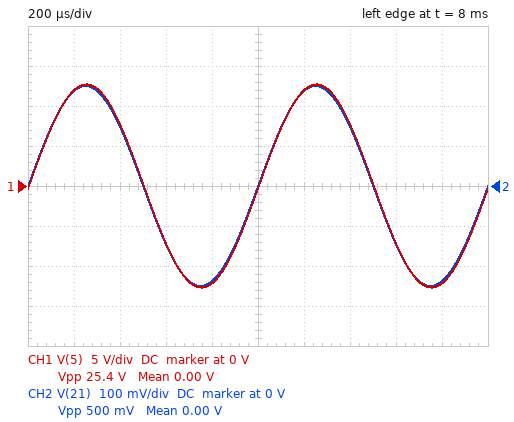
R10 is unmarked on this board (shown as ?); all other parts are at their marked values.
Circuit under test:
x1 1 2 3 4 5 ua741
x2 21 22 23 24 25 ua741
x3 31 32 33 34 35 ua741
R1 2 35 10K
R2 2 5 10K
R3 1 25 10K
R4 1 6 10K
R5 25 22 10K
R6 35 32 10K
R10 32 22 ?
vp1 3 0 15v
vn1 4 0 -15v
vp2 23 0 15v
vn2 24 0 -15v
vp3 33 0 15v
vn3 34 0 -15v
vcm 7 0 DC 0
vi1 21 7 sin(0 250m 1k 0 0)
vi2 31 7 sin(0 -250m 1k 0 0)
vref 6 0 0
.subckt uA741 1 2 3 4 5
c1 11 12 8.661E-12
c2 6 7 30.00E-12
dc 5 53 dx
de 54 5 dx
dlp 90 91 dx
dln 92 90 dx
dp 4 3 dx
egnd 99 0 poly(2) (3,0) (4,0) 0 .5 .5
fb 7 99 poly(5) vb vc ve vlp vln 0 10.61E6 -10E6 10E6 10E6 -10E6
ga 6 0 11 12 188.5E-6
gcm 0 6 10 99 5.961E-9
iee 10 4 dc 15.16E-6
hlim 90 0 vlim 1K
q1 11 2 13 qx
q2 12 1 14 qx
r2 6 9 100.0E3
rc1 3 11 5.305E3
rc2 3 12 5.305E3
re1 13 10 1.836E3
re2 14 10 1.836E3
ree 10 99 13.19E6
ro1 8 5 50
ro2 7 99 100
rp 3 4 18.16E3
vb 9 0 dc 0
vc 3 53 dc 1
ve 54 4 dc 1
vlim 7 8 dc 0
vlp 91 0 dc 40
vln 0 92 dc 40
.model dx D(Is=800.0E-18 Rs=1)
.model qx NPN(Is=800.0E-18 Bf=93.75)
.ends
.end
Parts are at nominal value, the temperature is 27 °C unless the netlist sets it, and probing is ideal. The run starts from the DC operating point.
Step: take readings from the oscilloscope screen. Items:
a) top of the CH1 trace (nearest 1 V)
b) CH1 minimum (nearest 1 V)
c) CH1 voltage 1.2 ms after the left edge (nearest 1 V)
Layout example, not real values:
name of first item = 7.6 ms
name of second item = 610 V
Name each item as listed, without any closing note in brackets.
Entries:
top of the CH1 trace = 13 V
CH1 minimum = -13 V
CH1 voltage 1.2 ms after the left edge = 12 V
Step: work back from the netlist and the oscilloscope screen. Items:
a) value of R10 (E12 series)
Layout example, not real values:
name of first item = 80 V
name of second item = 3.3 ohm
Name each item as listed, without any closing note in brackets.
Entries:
value of R10 = 820 Ω
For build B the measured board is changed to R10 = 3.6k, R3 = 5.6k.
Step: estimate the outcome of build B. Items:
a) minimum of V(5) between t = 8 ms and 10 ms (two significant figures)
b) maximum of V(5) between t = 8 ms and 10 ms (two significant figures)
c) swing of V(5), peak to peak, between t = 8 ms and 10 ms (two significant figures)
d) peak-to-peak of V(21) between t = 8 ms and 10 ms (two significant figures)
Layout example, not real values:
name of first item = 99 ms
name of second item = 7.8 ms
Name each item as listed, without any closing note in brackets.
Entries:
minimum of V(5) between t = 8 ms and 10 ms = -3.7 V
maximum of V(5) between t = 8 ms and 10 ms = 3.7 V
swing of V(5), peak to peak, between t = 8 ms and 10 ms = 7.5 V
peak-to-peak of V(21) between t = 8 ms and 10 ms = 500 mV
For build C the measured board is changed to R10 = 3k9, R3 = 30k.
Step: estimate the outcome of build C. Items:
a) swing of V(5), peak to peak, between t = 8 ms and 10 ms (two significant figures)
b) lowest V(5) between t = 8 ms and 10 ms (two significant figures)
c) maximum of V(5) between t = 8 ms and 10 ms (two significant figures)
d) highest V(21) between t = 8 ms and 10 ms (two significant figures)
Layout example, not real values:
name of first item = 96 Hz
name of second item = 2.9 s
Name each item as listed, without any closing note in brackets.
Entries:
swing of V(5), peak to peak, between t = 8 ms and 10 ms = 4.6 V
lowest V(5) between t = 8 ms and 10 ms = -2.3 V
maximum of V(5) between t = 8 ms and 10 ms = 2.3 V
highest V(21) between t = 8 ms and 10 ms = 250 mV
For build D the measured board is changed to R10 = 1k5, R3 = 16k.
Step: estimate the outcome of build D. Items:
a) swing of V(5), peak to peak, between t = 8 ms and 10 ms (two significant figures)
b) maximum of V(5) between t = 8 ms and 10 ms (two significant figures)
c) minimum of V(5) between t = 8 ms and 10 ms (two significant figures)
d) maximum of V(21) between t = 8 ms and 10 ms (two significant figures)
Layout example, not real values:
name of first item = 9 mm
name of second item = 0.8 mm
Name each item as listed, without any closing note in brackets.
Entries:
swing of V(5), peak to peak, between t = 8 ms and 10 ms = 13 V
maximum of V(5) between t = 8 ms and 10 ms = 6.3 V
minimum of V(5) between t = 8 ms and 10 ms = -6.3 V
maximum of V(21) between t = 8 ms and 10 ms = 250 mV
